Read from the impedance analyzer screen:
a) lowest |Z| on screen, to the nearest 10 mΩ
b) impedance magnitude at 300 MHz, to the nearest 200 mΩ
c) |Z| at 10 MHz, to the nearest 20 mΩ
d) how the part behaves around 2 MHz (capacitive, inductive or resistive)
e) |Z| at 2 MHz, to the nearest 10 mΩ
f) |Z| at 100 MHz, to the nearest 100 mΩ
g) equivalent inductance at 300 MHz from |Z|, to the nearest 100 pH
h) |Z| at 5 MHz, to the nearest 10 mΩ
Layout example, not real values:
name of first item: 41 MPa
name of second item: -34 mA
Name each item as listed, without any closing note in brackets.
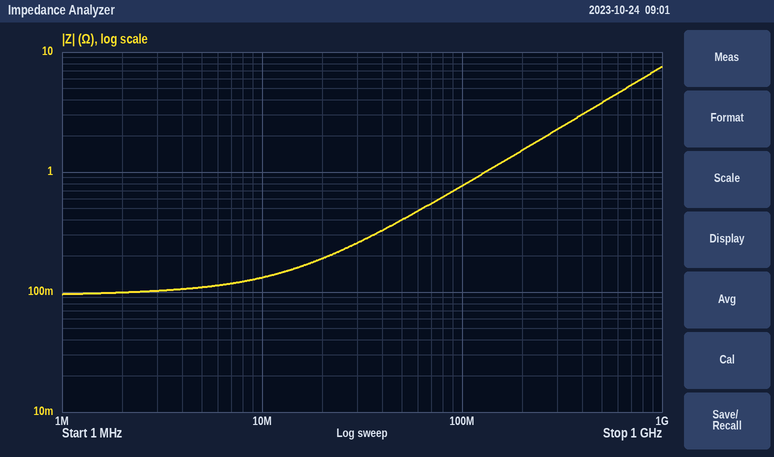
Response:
lowest |Z| on screen, to the nearest 10 mΩ: 100 mΩ
impedance magnitude at 300 MHz, to the nearest 200 mΩ: 2.2 Ω
|Z| at 10 MHz, to the nearest 20 mΩ: 140 mΩ
how the part behaves around 2 MHz: resistive
|Z| at 2 MHz, to the nearest 10 mΩ: 100 mΩ
|Z| at 100 MHz, to the nearest 100 mΩ: 800 mΩ
equivalent inductance at 300 MHz from |Z|, to the nearest 100 pH: 1.2 nH
|Z| at 5 MHz, to the nearest 10 mΩ: 110 mΩ
